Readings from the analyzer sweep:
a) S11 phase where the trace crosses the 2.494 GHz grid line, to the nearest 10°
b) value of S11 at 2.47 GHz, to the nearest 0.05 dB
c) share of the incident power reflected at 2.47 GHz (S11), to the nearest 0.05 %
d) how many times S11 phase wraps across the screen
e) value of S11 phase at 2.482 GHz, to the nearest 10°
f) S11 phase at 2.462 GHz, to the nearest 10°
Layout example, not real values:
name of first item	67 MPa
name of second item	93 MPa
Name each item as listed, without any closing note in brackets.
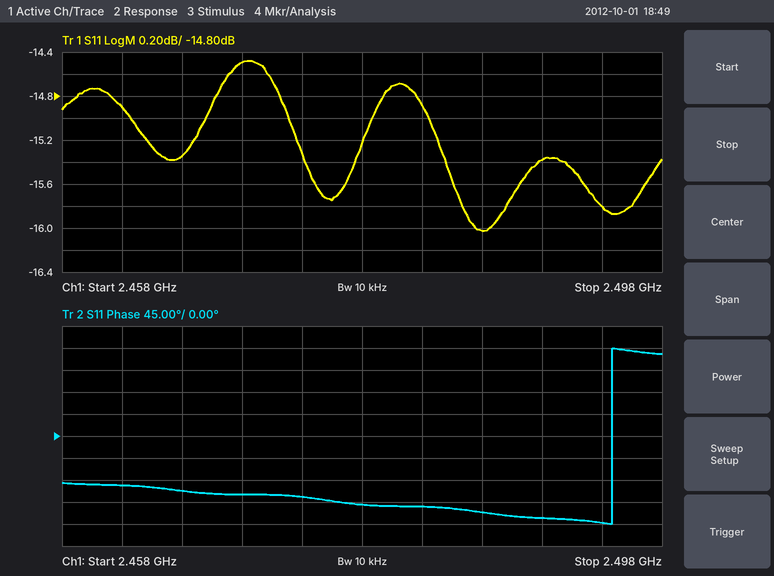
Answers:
S11 phase where the trace crosses the 2.494 GHz grid line, to the nearest 10°	-180°
value of S11 at 2.47 GHz, to the nearest 0.05 dB	-14.50 dB
share of the incident power reflected at 2.47 GHz (S11), to the nearest 0.05 %	3.55 %
how many times S11 phase wraps across the screen	1
value of S11 phase at 2.482 GHz, to the nearest 10°	-140°
S11 phase at 2.462 GHz, to the nearest 10°	-100°
